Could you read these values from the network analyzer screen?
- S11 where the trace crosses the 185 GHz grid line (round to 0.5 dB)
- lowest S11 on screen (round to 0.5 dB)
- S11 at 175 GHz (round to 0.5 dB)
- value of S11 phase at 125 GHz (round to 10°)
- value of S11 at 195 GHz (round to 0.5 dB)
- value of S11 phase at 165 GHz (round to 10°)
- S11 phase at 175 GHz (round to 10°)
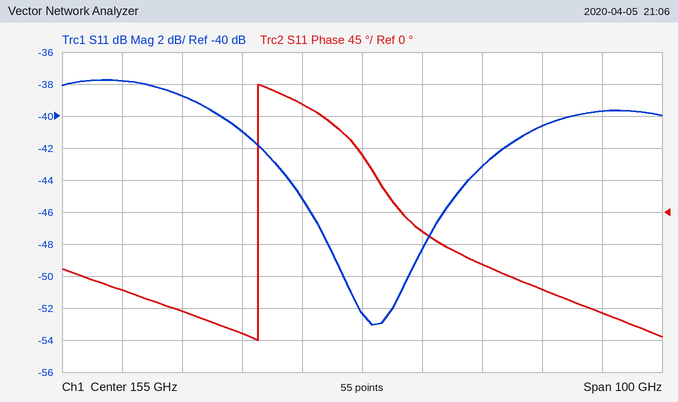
-40.5 dB
-53.0 dB
-43.0 dB
-140°
-39.5 dB
-30°
-70°
